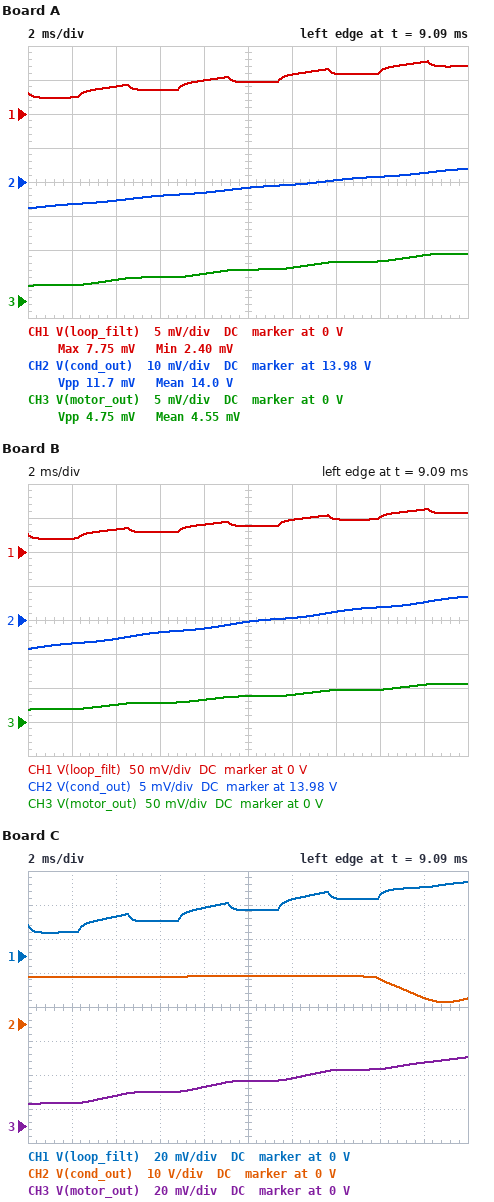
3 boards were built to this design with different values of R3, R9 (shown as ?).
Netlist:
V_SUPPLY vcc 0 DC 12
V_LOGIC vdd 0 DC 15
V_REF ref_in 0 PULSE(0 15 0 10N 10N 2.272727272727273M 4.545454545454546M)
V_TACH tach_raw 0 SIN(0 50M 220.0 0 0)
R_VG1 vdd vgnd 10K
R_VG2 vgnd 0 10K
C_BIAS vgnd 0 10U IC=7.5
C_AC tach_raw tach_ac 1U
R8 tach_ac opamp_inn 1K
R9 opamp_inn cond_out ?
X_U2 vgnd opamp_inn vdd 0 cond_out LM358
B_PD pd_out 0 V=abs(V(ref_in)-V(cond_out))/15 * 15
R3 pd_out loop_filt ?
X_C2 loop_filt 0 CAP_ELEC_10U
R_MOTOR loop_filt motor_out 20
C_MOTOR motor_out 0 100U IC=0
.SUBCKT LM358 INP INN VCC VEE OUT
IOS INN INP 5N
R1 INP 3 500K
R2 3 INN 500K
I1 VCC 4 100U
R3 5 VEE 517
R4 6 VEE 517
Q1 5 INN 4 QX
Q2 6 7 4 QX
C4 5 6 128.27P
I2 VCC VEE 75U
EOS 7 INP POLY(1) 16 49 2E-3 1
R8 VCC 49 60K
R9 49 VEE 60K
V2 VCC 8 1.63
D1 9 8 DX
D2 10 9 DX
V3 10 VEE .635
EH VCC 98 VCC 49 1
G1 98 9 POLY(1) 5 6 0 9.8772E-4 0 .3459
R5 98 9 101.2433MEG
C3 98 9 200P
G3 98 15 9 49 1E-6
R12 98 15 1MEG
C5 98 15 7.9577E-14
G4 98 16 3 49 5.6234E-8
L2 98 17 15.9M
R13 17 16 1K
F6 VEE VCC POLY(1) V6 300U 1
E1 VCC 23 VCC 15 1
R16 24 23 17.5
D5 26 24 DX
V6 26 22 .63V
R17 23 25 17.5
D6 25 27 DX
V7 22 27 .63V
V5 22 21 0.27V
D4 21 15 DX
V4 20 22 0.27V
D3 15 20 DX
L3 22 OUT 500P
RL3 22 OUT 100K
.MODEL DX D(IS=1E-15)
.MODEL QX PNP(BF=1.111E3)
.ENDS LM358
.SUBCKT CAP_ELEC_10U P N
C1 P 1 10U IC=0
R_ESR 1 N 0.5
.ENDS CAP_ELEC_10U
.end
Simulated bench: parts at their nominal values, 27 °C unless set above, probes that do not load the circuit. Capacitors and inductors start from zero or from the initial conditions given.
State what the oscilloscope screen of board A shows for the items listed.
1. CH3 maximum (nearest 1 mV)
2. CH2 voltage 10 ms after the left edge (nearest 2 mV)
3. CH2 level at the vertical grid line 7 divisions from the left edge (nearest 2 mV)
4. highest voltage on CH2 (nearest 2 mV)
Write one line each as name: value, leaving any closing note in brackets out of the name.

CH3 maximum: 7 mV
CH2 voltage 10 ms after the left edge: 13.978 V
CH2 level at the vertical grid line 7 divisions from the left edge: 13.980 V
highest voltage on CH2: 13.984 V
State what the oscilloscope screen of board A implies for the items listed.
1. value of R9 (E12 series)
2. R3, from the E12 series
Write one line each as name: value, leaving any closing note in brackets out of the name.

value of R9: 47 kΩ
R3, from the E12 series: 270 kΩ
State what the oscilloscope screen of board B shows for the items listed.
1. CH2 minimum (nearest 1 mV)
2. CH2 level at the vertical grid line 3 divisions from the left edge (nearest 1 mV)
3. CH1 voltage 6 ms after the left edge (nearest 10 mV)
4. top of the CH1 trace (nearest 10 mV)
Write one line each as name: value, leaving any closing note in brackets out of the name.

CH2 minimum: 13.981 V
CH2 level at the vertical grid line 3 divisions from the left edge: 13.983 V
CH1 voltage 6 ms after the left edge: 30 mV
top of the CH1 trace: 60 mV
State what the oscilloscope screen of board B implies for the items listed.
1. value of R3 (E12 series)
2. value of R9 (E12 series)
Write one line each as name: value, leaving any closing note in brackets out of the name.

value of R3: 33 kΩ
value of R9: 68 kΩ
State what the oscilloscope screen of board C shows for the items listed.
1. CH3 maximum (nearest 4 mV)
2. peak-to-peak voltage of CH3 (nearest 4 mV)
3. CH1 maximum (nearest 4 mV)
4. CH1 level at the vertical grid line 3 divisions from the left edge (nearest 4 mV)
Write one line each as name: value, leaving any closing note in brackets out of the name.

CH3 maximum: 40 mV
peak-to-peak voltage of CH3: 28 mV
CH1 maximum: 44 mV
CH1 level at the vertical grid line 3 divisions from the left edge: 20 mV
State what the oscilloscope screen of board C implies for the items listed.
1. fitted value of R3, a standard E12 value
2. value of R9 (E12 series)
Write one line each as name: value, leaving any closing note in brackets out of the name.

fitted value of R3, a standard E12 value: 47 kΩ
value of R9: 33 kΩ
